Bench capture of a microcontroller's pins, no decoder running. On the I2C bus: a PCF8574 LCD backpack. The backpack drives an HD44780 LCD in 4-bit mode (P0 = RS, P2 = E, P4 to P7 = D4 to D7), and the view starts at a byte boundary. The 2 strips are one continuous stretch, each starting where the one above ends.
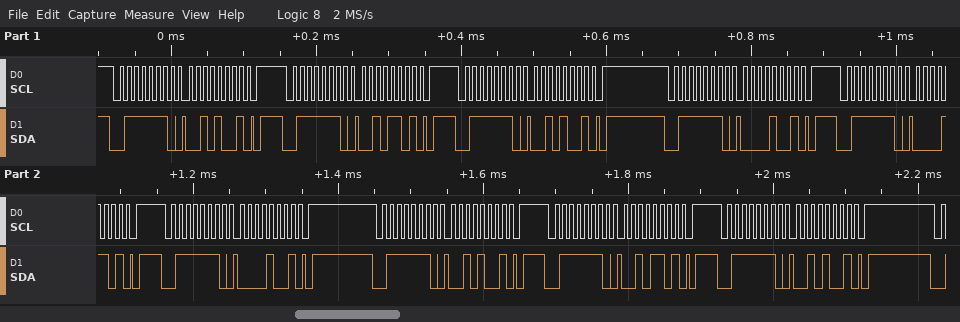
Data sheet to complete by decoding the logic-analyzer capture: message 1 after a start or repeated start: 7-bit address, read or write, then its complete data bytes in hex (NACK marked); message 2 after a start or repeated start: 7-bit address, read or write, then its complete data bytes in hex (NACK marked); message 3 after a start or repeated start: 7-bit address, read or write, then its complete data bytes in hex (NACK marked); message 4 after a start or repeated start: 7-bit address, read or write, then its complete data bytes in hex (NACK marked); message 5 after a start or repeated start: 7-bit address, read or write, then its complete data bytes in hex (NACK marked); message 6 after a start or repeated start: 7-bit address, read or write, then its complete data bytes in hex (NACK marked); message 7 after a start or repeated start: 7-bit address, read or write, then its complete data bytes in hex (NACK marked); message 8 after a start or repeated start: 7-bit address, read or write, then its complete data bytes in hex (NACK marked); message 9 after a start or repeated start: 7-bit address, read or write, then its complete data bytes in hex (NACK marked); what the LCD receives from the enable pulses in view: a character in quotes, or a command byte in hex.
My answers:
0x3F write: 29
0x3F write: 2D
0x3F write: 29
0x3F write: 09
0x3F write: 0D
0x3F write: 09
0x3F write: 29
0x3F write: 2D
0x3F write: 29
' '
